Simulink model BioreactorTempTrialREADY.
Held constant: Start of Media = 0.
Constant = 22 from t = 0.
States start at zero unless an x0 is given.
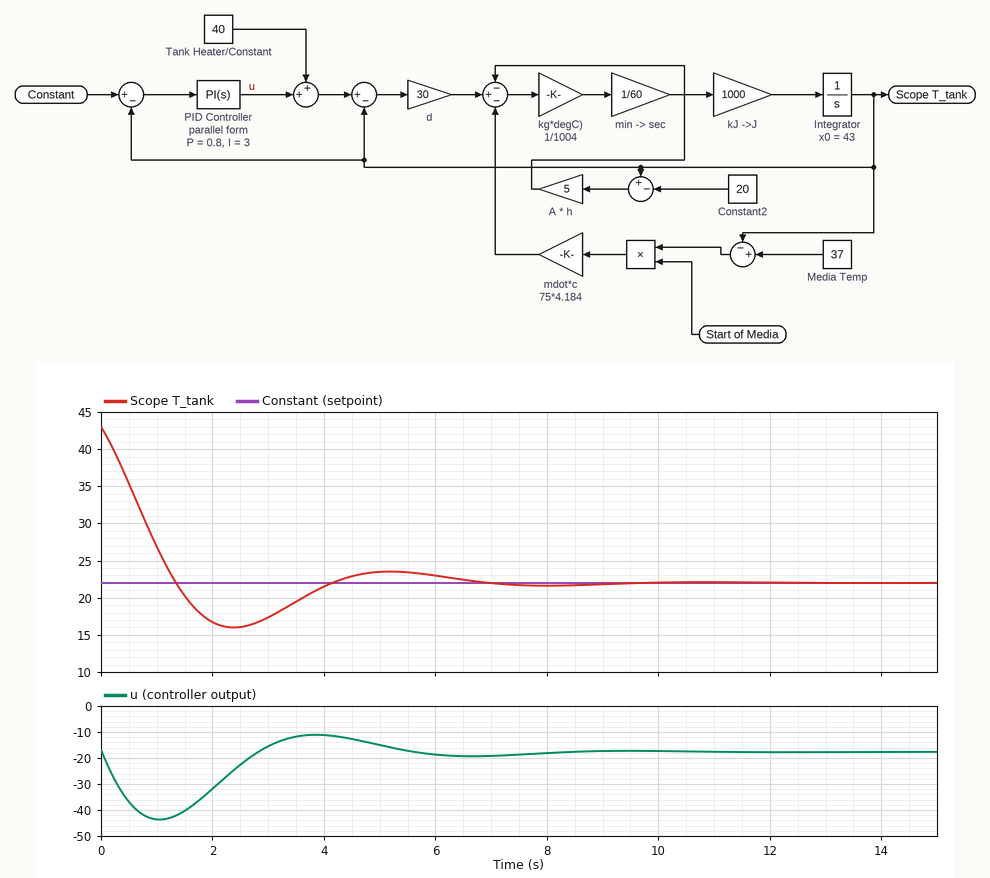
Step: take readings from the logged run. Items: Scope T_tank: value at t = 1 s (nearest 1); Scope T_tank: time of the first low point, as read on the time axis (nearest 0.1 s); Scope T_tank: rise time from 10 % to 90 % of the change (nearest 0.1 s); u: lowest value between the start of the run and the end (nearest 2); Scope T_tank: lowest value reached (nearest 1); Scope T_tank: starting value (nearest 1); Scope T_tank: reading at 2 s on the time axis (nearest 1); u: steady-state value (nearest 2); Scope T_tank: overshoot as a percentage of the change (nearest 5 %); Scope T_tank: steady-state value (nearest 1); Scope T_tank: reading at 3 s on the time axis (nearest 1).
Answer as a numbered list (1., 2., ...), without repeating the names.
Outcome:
1. 27
2. 2.4 s
3. 1.0 s
4. -44
5. 16
6. 43
7. 17
8. -18
9. 30 %
10. 22
11. 17
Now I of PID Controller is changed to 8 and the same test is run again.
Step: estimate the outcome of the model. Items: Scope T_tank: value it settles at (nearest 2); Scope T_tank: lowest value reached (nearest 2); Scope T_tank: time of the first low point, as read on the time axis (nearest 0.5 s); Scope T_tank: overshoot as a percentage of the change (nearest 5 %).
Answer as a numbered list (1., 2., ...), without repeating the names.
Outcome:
1. 22
2. 12
3. 1.5 s
4. 45 %
